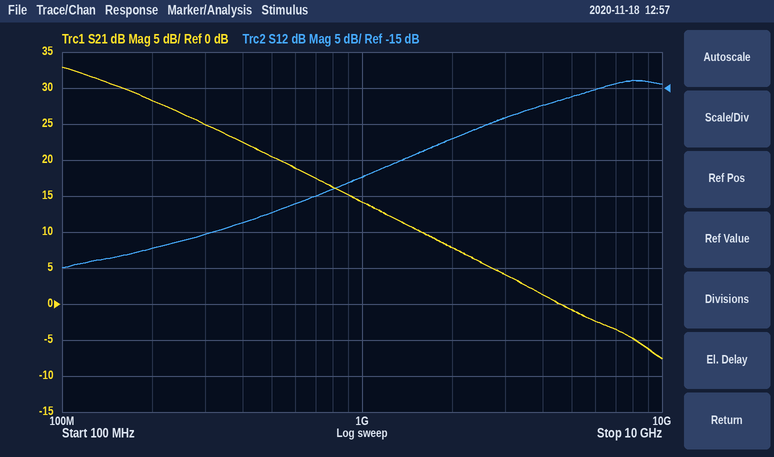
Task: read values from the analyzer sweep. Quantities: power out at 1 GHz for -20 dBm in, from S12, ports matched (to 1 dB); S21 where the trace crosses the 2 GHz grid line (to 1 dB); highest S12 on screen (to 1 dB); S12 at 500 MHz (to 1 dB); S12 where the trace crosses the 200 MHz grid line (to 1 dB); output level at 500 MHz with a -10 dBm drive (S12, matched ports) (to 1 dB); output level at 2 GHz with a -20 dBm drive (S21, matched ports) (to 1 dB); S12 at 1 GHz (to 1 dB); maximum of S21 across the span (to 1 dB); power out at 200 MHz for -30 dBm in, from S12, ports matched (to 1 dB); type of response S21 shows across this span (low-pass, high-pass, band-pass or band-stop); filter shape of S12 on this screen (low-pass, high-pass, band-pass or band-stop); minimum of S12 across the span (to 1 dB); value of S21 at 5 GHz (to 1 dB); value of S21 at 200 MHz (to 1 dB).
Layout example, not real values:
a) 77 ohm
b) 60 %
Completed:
a) -47 dBm
b) 8 dB
c) -14 dB
d) -32 dB
e) -37 dB
f) -42 dBm
g) -12 dBm
h) -27 dB
i) 33 dB
j) -67 dBm
k) low-pass
l) high-pass
m) -40 dB
n) -1 dB
o) 28 dB
